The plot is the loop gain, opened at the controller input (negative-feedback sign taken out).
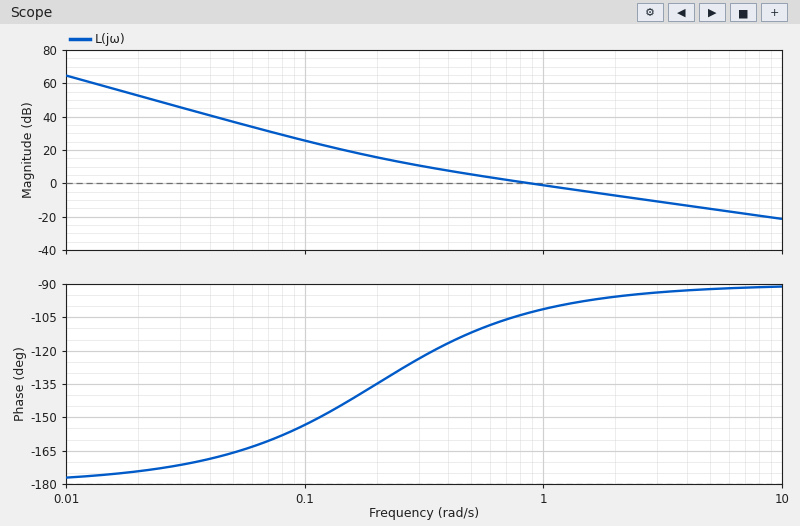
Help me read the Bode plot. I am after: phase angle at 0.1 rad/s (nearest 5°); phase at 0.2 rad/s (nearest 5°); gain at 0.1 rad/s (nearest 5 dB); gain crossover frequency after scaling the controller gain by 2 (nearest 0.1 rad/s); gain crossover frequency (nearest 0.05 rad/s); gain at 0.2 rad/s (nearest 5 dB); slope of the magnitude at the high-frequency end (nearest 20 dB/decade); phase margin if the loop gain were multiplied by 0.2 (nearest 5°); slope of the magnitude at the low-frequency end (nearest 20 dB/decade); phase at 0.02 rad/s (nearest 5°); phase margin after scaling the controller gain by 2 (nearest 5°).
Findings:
-155°
-135°
25 dB
1.7 rad/s
0.90 rad/s
15 dB
-20 dB/decade
50°
-40 dB/decade
-175°
85°
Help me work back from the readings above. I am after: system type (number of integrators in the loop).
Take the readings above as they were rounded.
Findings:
2
